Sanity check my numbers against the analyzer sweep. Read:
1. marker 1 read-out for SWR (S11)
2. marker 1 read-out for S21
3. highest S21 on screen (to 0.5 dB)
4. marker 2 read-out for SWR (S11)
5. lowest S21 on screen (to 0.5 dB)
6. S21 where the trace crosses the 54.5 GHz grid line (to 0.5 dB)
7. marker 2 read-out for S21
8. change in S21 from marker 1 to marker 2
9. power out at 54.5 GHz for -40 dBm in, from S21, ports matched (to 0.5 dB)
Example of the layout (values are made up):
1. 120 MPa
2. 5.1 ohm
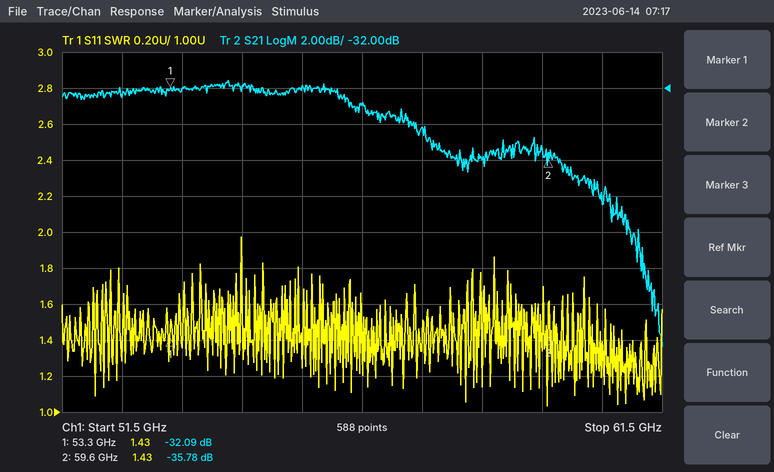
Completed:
1. 1.43
2. -32.09 dB
3. -31.5 dB
4. 1.43
5. -46.5 dB
6. -32.0 dB
7. -35.78 dB
8. -3.69 dB
9. -72.0 dBm
